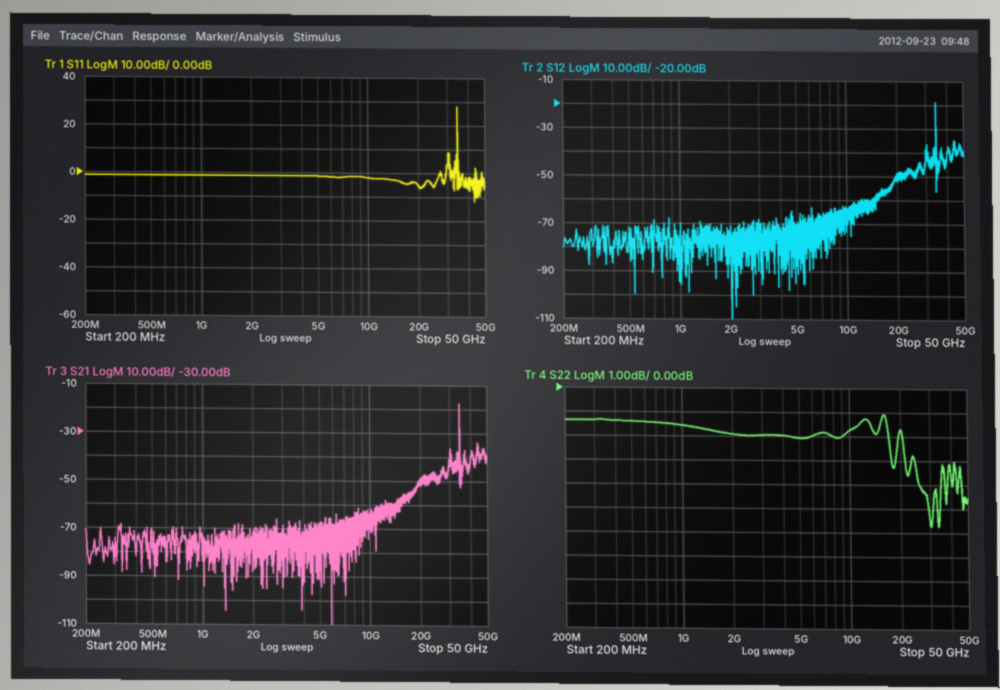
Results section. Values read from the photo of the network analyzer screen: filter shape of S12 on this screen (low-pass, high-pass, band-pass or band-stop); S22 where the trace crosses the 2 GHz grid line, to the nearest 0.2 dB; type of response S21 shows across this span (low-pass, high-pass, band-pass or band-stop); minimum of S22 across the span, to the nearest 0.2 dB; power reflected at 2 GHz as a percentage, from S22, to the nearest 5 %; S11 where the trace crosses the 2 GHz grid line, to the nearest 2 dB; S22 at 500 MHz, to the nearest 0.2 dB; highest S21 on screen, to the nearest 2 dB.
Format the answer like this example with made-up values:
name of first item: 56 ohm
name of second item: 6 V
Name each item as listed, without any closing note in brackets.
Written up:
filter shape of S12 on this screen: band-pass
S22 where the trace crosses the 2 GHz grid line, to the nearest 0.2 dB: -2.0 dB
type of response S21 shows across this span: band-pass
minimum of S22 across the span, to the nearest 0.2 dB: -5.8 dB
power reflected at 2 GHz as a percentage, from S22, to the nearest 5 %: 65 %
S11 where the trace crosses the 2 GHz grid line, to the nearest 2 dB: -2 dB
S22 at 500 MHz, to the nearest 0.2 dB: -1.4 dB
highest S21 on screen, to the nearest 2 dB: -18 dB
